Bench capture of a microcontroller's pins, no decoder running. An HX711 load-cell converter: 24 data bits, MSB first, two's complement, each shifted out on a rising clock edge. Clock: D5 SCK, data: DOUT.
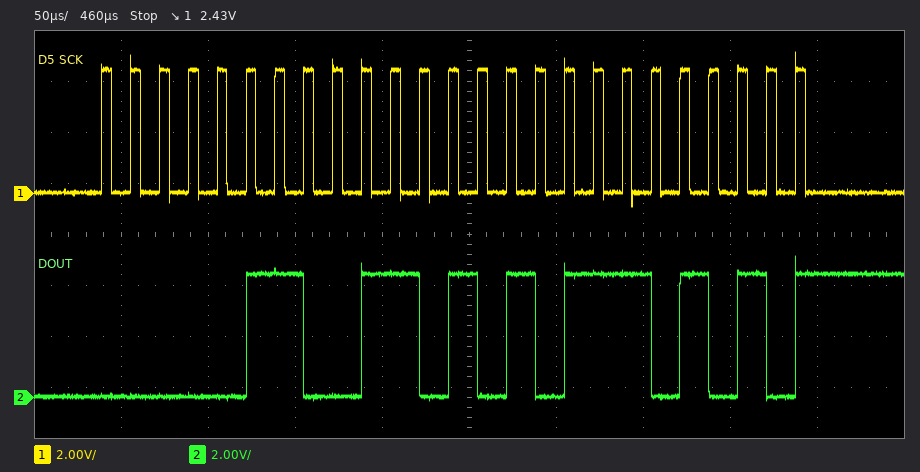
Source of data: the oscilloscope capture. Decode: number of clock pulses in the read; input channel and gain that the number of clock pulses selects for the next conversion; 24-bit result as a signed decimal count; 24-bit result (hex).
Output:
25
channel A, gain 128
420586
0x066AEA
